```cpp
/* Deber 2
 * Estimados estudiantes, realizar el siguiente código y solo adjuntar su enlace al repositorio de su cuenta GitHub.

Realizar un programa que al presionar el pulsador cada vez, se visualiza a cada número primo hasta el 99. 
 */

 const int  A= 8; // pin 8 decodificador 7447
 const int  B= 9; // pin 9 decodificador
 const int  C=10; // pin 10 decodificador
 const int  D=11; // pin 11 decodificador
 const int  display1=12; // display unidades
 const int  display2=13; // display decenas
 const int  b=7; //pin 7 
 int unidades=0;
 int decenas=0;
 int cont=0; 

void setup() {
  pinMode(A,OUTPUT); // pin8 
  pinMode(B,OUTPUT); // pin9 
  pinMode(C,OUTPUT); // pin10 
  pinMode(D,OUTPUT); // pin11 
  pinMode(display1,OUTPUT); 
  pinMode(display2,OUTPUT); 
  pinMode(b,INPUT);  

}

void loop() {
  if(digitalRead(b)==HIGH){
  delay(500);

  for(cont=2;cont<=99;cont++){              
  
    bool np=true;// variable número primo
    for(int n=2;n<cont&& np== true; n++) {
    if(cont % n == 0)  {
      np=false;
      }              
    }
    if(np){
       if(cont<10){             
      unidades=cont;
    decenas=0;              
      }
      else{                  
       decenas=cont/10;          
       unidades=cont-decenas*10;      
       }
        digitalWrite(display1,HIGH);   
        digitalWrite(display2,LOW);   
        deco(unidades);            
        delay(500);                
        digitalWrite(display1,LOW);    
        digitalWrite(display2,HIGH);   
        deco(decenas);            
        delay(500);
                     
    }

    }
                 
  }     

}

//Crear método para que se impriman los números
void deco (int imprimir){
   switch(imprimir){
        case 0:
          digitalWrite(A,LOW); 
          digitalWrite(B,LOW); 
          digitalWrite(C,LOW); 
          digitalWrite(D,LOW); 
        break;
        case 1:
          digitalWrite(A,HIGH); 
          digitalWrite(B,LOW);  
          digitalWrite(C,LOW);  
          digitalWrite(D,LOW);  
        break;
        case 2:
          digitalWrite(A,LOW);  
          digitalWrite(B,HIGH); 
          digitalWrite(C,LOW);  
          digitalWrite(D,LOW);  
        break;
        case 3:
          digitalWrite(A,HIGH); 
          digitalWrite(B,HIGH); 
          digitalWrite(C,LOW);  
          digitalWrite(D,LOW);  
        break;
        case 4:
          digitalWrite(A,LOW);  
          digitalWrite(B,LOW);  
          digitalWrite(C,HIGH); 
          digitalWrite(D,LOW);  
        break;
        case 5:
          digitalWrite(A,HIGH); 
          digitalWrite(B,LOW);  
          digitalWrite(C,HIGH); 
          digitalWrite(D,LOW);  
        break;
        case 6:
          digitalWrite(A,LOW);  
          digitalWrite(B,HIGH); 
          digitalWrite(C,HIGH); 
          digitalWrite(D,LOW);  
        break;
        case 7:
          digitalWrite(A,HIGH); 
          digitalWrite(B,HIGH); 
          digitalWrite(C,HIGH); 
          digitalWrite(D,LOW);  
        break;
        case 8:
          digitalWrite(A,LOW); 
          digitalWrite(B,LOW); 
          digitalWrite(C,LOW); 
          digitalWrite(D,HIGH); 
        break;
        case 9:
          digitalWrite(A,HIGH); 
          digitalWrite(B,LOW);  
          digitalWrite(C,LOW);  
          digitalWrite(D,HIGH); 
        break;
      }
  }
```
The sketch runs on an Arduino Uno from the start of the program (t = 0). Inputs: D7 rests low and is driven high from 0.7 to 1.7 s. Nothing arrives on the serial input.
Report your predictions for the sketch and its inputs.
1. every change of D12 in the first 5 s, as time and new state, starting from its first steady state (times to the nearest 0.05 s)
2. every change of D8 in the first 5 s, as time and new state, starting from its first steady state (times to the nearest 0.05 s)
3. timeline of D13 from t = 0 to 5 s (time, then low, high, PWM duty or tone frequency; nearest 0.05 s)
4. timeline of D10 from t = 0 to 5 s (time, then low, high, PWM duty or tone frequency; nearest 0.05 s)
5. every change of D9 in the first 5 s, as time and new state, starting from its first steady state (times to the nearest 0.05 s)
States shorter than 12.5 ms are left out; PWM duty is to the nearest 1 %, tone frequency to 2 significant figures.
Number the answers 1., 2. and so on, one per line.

1. 0 s low; 1.2 s high; 1.7 s low; 2.2 s high; 2.7 s low; 3.2 s high; 3.7 s low; 4.2 s high; 4.7 s low
2. 0 s low; 2.2 s high; 2.7 s low; 3.2 s high; 3.7 s low; 4.2 s high; 4.7 s low
3. 0 s low; 1.7 s high; 2.2 s low; 2.7 s high; 3.2 s low; 3.7 s high; 4.2 s low; 4.7 s high
4. 0 s low; 3.2 s high; 3.7 s low; 4.2 s high; 4.7 s low
5. 0 s low; 1.2 s high; 1.7 s low; 2.2 s high; 2.7 s low; 4.2 s high; 4.7 s low
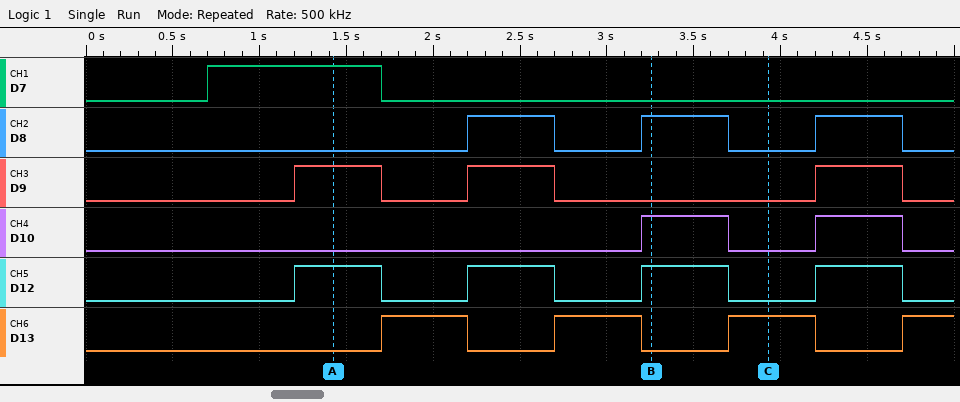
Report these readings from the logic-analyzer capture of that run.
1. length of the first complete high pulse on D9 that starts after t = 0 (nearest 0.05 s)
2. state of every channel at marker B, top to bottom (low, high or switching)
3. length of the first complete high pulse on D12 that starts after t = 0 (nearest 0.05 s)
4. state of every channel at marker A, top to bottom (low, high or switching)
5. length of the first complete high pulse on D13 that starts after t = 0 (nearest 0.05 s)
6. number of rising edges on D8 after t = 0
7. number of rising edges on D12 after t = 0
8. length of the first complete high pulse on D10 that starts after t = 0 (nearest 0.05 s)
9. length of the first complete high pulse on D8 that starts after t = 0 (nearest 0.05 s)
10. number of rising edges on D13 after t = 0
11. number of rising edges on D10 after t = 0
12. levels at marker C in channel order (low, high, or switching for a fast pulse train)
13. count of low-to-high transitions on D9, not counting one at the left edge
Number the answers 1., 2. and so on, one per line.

1. 0.50 s
2. D7 low, D8 high, D9 low, D10 high, D12 high, D13 low
3. 0.50 s
4. D7 high, D8 low, D9 high, D10 low, D12 high, D13 low
5. 0.50 s
6. 3
7. 4
8. 0.50 s
9. 0.50 s
10. 4
11. 2
12. D7 low, D8 low, D9 low, D10 low, D12 low, D13 high
13. 3
